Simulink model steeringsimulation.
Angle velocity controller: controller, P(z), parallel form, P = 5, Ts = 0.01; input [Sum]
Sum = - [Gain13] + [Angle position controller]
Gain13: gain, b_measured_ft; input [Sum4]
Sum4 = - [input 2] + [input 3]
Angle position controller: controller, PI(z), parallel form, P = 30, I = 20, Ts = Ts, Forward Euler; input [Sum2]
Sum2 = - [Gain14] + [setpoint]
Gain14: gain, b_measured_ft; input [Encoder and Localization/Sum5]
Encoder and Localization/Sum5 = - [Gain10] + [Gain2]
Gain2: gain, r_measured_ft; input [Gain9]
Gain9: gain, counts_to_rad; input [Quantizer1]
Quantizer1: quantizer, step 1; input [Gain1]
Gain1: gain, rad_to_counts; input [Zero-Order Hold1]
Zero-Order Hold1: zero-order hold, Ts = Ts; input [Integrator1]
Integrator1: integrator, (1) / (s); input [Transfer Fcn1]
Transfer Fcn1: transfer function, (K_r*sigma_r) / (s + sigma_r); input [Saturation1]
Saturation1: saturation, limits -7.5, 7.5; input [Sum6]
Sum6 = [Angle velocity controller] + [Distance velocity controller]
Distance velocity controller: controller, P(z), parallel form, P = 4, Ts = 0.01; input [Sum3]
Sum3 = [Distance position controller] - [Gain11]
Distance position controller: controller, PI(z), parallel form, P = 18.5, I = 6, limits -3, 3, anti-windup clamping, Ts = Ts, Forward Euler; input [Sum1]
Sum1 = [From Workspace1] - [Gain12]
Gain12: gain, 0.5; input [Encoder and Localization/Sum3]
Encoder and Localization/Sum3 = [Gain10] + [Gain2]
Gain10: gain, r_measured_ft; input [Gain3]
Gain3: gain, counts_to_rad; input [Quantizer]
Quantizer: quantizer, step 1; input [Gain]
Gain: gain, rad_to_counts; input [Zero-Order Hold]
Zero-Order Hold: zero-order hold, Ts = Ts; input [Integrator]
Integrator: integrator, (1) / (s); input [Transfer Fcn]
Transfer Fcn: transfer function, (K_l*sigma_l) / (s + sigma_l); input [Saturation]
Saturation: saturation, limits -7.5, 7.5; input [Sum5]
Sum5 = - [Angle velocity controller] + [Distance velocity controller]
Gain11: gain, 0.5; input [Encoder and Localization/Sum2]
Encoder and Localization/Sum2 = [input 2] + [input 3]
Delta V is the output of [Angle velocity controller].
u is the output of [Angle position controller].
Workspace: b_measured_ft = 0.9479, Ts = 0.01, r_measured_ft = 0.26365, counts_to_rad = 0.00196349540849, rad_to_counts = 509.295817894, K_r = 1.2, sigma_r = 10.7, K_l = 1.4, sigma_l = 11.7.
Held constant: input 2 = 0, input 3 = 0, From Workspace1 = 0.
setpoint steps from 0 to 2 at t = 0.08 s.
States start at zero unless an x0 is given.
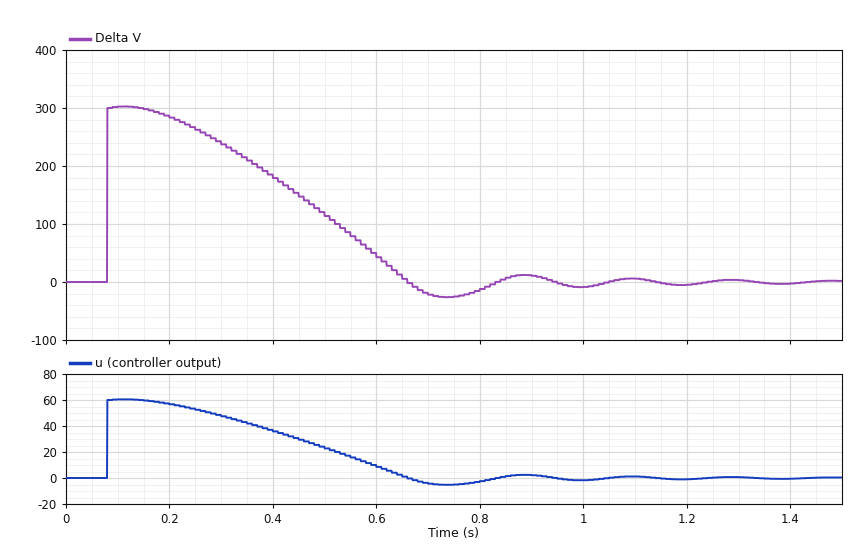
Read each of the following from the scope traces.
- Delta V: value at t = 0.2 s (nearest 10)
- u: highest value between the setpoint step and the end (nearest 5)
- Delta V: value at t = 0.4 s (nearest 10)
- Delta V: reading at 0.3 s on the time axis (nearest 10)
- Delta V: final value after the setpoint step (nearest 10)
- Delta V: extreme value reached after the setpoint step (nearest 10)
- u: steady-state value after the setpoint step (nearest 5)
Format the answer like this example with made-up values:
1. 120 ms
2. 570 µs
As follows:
1. 280
2. 60
3. 180
4. 240
5. 0
6. 300
7. 0
